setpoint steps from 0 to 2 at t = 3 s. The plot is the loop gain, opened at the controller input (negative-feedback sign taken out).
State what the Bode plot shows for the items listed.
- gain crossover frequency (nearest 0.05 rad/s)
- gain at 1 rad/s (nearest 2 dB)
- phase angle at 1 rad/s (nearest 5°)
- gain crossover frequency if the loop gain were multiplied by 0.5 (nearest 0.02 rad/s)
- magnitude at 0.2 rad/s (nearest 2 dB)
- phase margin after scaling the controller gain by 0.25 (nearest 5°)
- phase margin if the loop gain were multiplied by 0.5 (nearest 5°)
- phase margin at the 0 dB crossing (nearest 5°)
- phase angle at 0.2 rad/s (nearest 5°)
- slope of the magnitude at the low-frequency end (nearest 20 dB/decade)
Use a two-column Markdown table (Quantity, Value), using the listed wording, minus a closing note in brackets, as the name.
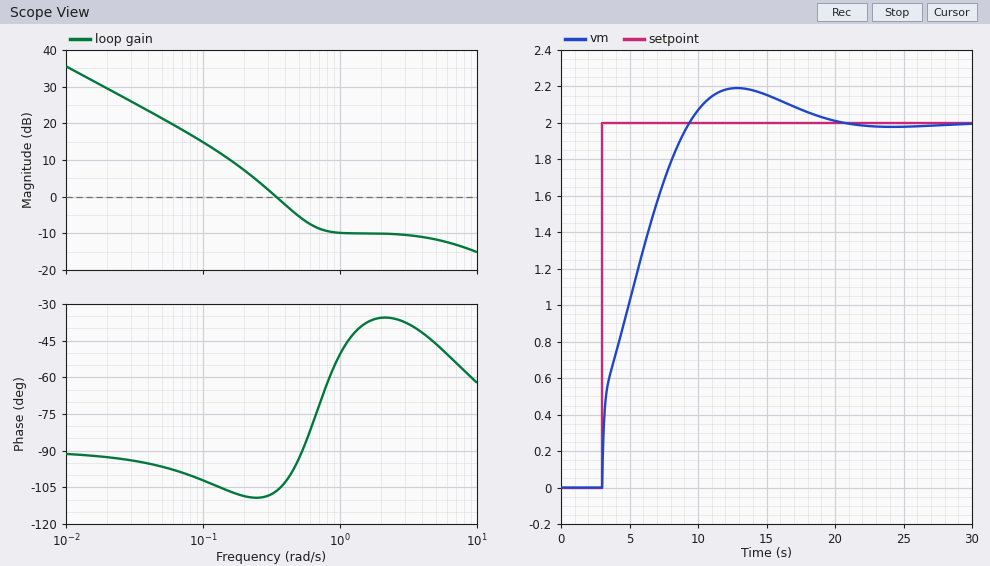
| Quantity | Value |
|---|---|
| gain crossover frequency | 0.35 rad/s |
| gain at 1 rad/s | -10 dB |
| phase angle at 1 rad/s | -50° |
| gain crossover frequency if the loop gain were multiplied by 0.5 | 0.22 rad/s |
| magnitude at 0.2 rad/s | 8 dB |
| phase margin after scaling the controller gain by 0.25 | 75° |
| phase margin if the loop gain were multiplied by 0.5 | 70° |
| phase margin at the 0 dB crossing | 75° |
| phase angle at 0.2 rad/s | -110° |
| slope of the magnitude at the low-frequency end | -20 dB/decade |
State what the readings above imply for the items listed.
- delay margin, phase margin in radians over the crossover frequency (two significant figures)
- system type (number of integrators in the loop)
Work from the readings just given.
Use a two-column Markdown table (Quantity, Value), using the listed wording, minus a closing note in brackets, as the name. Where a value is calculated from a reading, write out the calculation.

| Quantity | Value |
|---|---|
| delay margin, phase margin in radians over the crossover frequency | 75 × π / 180 / 0.35 = 3.7 s |
| system type | 1 |
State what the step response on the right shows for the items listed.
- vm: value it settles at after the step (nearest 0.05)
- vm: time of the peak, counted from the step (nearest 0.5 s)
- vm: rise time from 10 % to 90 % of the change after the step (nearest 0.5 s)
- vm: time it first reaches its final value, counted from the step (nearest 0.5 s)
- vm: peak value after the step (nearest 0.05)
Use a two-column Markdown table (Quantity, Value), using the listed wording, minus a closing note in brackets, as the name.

| Quantity | Value |
|---|---|
| vm: value it settles at after the step | 2.00 |
| vm: time of the peak, counted from the step | 10.0 s |
| vm: rise time from 10 % to 90 % of the change after the step | 5.0 s |
| vm: time it first reaches its final value, counted from the step | 6.5 s |
| vm: peak value after the step | 2.20 |
